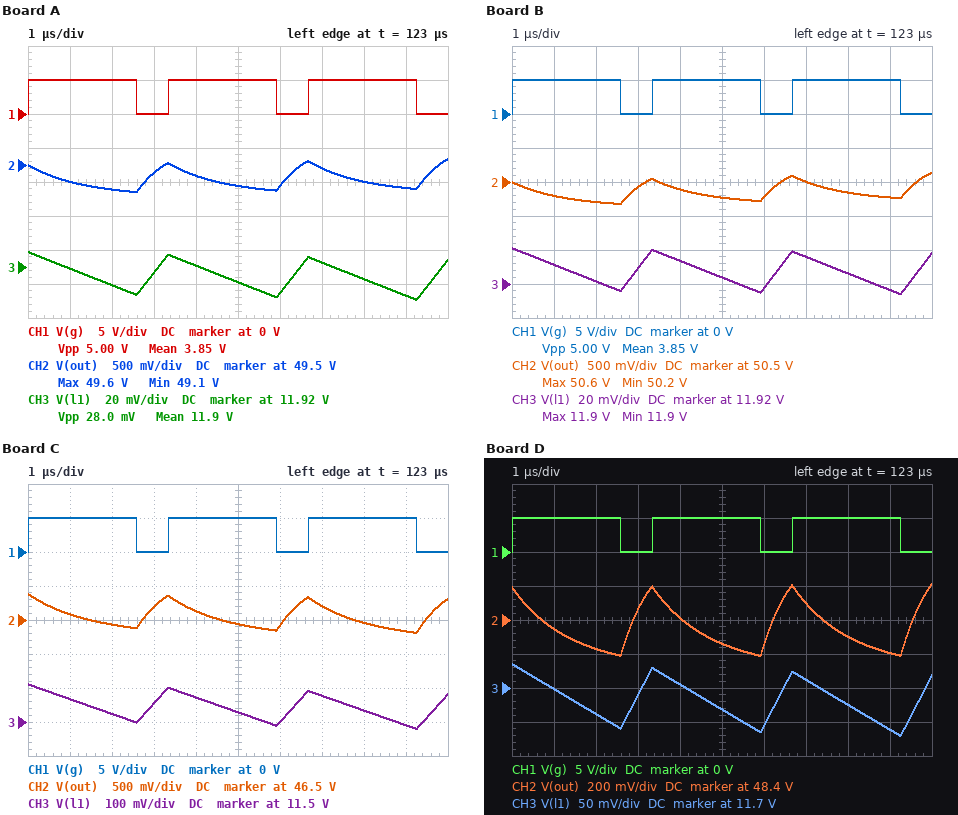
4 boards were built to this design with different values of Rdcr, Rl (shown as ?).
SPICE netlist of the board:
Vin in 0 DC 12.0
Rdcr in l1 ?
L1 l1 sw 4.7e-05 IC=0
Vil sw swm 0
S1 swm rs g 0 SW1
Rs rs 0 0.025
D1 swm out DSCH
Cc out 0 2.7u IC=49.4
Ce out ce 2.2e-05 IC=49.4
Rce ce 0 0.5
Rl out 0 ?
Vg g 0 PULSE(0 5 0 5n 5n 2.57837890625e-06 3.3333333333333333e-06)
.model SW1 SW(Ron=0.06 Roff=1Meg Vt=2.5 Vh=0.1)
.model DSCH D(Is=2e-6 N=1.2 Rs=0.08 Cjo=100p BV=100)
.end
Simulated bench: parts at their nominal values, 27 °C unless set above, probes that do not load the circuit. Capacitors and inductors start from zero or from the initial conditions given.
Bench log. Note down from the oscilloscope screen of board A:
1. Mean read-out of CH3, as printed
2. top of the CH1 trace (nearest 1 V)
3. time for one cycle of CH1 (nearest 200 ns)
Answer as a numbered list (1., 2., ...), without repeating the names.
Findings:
1. 11.9 V
2. 5 V
3. 3.4 µs
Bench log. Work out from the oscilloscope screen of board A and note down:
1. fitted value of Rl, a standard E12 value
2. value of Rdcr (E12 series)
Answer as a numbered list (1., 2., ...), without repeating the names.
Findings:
1. 150 Ω
2. 0.039 Ω
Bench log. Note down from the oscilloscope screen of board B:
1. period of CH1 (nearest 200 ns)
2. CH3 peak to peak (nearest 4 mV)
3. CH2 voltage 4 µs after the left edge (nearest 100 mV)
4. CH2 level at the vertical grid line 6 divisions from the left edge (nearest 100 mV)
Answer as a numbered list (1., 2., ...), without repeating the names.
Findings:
1. 3.4 µs
2. 28 mV
3. 50.4 V
4. 50.3 V
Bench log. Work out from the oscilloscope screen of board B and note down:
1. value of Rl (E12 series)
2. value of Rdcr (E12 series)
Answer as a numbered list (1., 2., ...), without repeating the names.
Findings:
1. 470 Ω
2. 0.039 Ω
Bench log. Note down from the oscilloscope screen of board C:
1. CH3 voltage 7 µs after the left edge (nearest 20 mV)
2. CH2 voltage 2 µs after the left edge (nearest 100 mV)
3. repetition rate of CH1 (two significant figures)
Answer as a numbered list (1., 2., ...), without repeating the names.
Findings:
1. 11.58 V
2. 46.4 V
3. 300 kHz
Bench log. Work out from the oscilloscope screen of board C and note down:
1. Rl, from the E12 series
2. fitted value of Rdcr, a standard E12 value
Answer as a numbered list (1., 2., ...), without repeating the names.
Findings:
1. 56 Ω
2. 0.18 Ω
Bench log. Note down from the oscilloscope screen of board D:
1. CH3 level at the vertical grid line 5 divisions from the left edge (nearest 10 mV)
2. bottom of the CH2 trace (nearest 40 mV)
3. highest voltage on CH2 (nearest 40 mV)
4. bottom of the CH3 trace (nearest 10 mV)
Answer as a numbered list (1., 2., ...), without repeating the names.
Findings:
1. 11.67 V
2. 48.20 V
3. 48.60 V
4. 11.63 V
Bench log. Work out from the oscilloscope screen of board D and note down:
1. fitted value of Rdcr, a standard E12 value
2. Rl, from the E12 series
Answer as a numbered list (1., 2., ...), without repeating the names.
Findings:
1. 0.15 Ω
2. 100 Ω
